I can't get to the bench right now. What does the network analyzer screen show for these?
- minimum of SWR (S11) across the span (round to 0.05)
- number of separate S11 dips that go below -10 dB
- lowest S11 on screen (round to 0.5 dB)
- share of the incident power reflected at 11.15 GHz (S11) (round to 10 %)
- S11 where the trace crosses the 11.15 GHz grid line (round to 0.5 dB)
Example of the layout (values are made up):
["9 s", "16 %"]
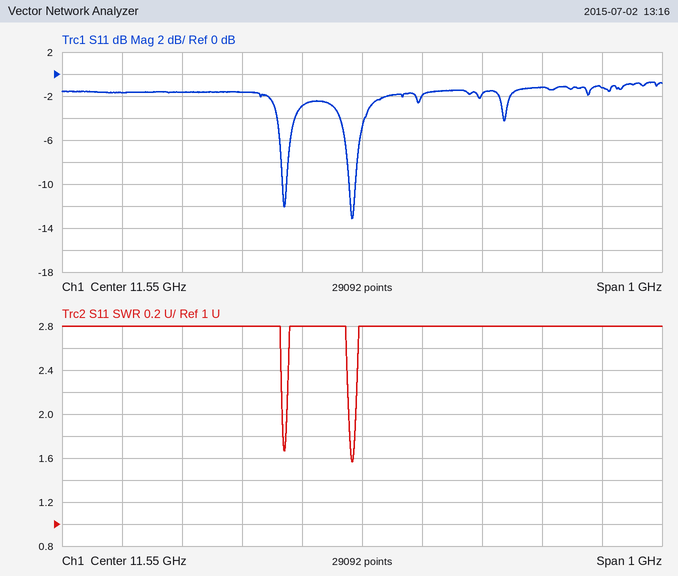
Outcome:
["1.55", "2", "-13.0 dB", "70 %", "-1.5 dB"]
